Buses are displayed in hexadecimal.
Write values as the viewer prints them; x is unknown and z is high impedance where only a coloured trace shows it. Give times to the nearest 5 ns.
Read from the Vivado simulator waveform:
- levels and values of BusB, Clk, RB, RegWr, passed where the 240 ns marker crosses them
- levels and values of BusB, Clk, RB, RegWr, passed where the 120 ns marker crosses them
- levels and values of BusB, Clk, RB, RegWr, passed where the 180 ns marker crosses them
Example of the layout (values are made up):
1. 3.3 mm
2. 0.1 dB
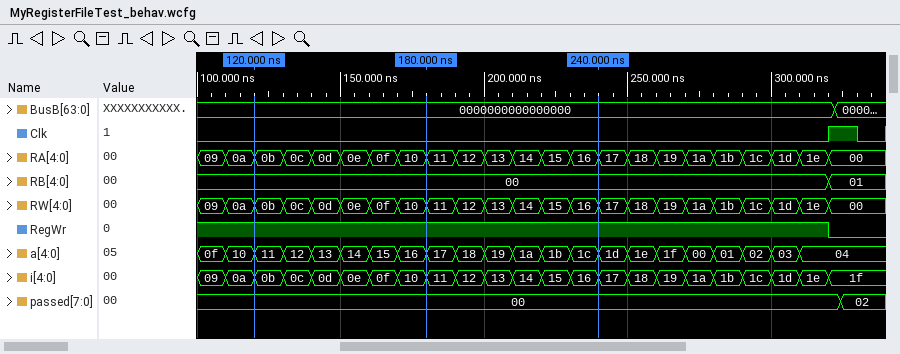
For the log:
1. BusB=0000000000000000, Clk=0, RB=00, RegWr=1, passed=00
2. BusB=0000000000000000, Clk=0, RB=00, RegWr=1, passed=00
3. BusB=0000000000000000, Clk=0, RB=00, RegWr=1, passed=00
